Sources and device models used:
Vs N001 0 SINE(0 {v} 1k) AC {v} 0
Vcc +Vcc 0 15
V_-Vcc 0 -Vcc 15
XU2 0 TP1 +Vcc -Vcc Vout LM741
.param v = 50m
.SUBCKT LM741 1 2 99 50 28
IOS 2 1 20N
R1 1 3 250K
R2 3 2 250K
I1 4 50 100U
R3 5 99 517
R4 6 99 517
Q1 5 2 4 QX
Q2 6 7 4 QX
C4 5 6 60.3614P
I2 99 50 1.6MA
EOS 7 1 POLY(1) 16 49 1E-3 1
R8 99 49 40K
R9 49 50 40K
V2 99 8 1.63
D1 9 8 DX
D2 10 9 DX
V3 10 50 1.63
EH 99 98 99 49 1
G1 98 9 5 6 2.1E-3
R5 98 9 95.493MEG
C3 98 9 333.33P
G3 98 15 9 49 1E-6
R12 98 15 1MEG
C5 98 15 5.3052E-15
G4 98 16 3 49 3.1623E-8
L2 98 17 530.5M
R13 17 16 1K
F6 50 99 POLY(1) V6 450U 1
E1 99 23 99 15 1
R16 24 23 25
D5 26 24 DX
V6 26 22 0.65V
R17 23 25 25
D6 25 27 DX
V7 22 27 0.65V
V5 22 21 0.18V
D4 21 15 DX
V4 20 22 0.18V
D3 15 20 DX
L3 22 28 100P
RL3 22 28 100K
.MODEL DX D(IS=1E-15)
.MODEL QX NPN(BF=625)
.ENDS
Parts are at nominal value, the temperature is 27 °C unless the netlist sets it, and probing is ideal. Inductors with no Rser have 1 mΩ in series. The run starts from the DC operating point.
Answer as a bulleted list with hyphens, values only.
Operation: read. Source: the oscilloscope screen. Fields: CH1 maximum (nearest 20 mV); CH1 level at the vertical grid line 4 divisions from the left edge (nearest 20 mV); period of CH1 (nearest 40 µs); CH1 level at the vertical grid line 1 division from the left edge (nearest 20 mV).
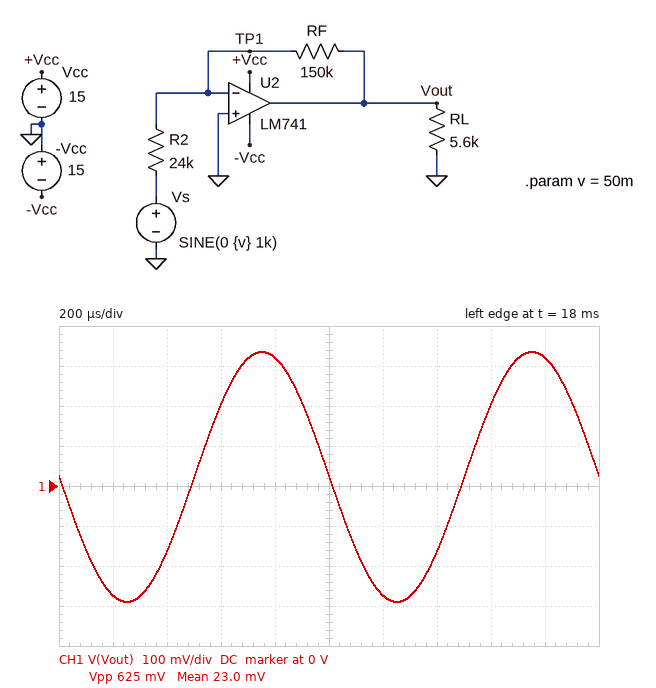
- 340 mV
- 320 mV
- 1.00 ms
- -280 mV
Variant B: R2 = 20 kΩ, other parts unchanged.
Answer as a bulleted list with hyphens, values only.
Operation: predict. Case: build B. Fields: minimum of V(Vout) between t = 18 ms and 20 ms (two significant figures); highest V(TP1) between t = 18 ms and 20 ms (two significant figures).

- -350 mV
- 1.4 mV
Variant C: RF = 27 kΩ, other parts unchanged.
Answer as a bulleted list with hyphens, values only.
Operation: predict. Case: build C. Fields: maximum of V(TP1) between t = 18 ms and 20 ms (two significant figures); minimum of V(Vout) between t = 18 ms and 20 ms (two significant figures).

- 1.1 mV
- -51 mV
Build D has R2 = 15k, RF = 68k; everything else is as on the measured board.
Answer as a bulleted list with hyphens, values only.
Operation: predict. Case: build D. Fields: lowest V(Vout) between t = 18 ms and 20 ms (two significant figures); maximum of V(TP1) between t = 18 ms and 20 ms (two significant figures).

- -210 mV
- 1.2 mV
